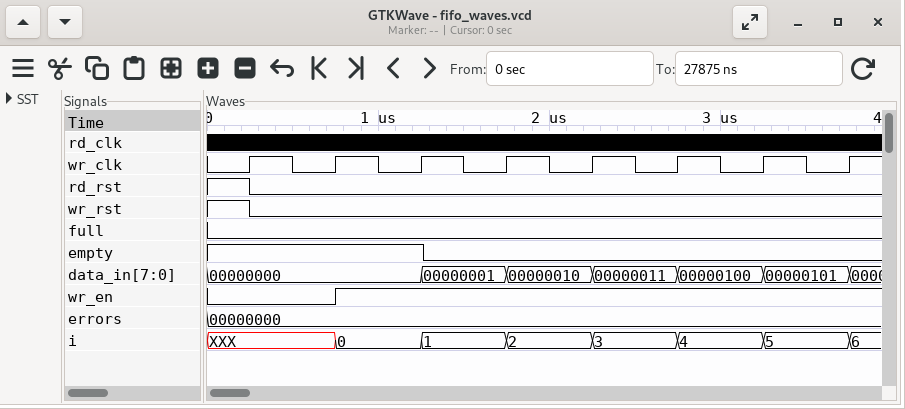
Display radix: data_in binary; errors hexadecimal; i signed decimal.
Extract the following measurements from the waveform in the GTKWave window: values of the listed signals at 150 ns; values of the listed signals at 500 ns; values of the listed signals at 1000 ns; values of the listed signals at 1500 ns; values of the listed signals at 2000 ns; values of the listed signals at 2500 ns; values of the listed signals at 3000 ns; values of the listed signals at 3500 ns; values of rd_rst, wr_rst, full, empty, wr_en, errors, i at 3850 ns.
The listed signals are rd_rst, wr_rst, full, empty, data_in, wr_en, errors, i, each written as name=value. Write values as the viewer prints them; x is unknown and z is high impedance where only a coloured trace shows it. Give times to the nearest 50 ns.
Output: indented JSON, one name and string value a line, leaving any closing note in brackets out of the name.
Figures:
{
  "values of the listed signals at 150 ns": "rd_rst=1, wr_rst=1, full=0, empty=1, data_in=00000000, wr_en=0, errors=00000000, i=XXX",
  "values of the listed signals at 500 ns": "rd_rst=0, wr_rst=0, full=0, empty=1, data_in=00000000, wr_en=0, errors=00000000, i=XXX",
  "values of the listed signals at 1000 ns": "rd_rst=0, wr_rst=0, full=0, empty=1, data_in=00000000, wr_en=1, errors=00000000, i=0",
  "values of the listed signals at 1500 ns": "rd_rst=0, wr_rst=0, full=0, empty=0, data_in=00000001, wr_en=1, errors=00000000, i=1",
  "values of the listed signals at 2000 ns": "rd_rst=0, wr_rst=0, full=0, empty=0, data_in=00000010, wr_en=1, errors=00000000, i=2",
  "values of the listed signals at 2500 ns": "rd_rst=0, wr_rst=0, full=0, empty=0, data_in=00000011, wr_en=1, errors=00000000, i=3",
  "values of the listed signals at 3000 ns": "rd_rst=0, wr_rst=0, full=0, empty=0, data_in=00000100, wr_en=1, errors=00000000, i=4",
  "values of the listed signals at 3500 ns": "rd_rst=0, wr_rst=0, full=0, empty=0, data_in=00000101, wr_en=1, errors=00000000, i=5",
  "values of rd_rst, wr_rst, full, empty, wr_en, errors, i at 3850 ns": "rd_rst=0, wr_rst=0, full=0, empty=0, wr_en=1, errors=00000000, i=6"
}
